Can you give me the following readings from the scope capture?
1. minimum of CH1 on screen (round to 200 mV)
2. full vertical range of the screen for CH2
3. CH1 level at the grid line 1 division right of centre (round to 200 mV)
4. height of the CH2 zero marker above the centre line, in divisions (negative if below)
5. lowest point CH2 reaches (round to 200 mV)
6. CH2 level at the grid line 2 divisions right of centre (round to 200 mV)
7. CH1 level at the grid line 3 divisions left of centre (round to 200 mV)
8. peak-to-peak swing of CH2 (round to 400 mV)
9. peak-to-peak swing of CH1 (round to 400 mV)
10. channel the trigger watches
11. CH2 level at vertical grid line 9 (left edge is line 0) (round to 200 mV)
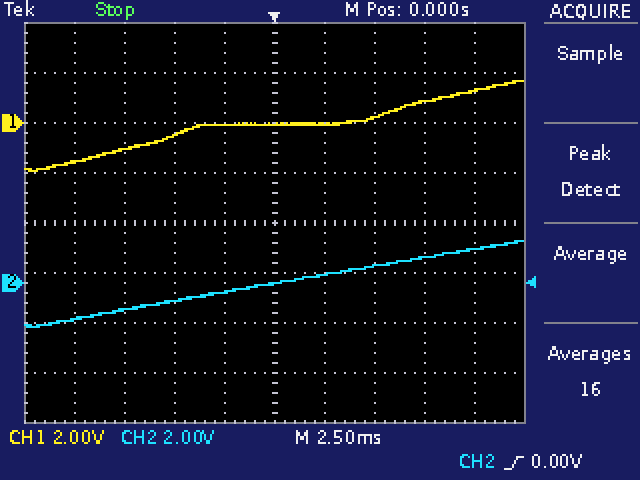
-2.0 V
16 V
0.0 V
-1.2 div
-1.8 V
600 mV
-1.0 V
3.6 V
3.6 V
CH2
1.4 V
